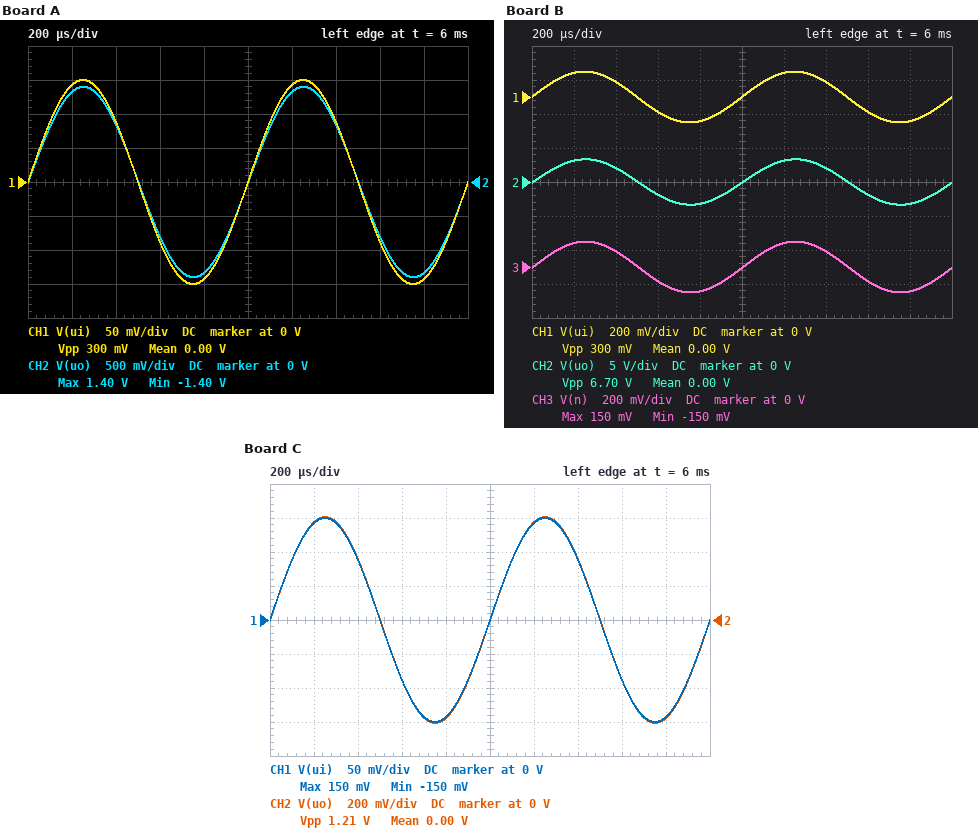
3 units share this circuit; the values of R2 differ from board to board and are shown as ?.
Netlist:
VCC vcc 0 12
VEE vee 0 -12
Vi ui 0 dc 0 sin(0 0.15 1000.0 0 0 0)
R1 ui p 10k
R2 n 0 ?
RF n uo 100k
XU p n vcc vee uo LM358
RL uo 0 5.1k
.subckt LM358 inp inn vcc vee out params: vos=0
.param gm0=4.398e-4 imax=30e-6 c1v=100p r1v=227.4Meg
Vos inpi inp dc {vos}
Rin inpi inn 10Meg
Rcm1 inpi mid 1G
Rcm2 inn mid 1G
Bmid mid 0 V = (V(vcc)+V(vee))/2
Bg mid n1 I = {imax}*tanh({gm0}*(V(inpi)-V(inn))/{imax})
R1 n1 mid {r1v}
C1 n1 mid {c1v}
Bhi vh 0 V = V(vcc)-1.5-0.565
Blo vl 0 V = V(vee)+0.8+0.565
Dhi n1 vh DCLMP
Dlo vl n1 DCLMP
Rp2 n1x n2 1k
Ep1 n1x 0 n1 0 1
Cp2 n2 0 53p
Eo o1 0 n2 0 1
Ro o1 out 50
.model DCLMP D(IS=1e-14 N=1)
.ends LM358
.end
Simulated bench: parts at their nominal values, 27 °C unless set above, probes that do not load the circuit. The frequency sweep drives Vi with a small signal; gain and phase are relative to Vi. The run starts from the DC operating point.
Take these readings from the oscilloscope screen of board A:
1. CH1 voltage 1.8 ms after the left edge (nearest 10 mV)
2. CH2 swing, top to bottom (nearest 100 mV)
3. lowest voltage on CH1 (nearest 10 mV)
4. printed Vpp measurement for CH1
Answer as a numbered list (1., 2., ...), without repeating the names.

1. -140 mV
2. 2.8 V
3. -150 mV
4. 300 mV
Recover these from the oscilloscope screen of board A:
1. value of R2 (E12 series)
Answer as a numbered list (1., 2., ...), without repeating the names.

1. 12 kΩ
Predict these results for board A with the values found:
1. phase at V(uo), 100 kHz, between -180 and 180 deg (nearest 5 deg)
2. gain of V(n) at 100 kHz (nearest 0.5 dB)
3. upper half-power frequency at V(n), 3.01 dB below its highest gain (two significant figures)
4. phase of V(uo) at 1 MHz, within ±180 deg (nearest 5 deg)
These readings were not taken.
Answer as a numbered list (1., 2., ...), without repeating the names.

1. -55 deg
2. -4.5 dB
3. 76 kHz
4. -105 deg
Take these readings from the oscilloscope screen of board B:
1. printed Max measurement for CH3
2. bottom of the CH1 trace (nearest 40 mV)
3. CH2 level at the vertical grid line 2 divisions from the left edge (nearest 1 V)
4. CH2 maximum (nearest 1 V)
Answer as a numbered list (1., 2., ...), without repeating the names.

1. 150 mV
2. -160 mV
3. 2 V
4. 3 V
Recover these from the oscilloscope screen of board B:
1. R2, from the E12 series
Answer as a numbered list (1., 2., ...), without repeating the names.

1. 4.7 kΩ
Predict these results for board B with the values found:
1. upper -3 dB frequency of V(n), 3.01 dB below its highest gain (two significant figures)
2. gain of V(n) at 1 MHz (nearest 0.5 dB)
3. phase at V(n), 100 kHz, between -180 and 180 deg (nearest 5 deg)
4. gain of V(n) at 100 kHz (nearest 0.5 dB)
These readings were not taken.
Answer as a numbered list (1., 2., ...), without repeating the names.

1. 31 kHz
2. -30.5 dB
3. -75 deg
4. -10.5 dB
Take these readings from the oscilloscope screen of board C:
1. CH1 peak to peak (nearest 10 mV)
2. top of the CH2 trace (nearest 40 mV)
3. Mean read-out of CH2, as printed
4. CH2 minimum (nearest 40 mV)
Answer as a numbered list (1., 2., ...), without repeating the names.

1. 300 mV
2. 600 mV
3. 0.00 V
4. -600 mV
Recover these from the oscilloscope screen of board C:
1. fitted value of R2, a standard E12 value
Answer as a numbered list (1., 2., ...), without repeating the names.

1. 33 kΩ
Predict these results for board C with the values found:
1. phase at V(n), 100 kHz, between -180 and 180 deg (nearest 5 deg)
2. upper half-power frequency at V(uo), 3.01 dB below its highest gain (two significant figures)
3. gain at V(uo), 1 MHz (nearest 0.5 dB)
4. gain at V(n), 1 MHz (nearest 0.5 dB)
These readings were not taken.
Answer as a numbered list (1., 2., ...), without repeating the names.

1. -30 deg
2. 180 kHz
3. -3.5 dB
4. -15.5 dB
